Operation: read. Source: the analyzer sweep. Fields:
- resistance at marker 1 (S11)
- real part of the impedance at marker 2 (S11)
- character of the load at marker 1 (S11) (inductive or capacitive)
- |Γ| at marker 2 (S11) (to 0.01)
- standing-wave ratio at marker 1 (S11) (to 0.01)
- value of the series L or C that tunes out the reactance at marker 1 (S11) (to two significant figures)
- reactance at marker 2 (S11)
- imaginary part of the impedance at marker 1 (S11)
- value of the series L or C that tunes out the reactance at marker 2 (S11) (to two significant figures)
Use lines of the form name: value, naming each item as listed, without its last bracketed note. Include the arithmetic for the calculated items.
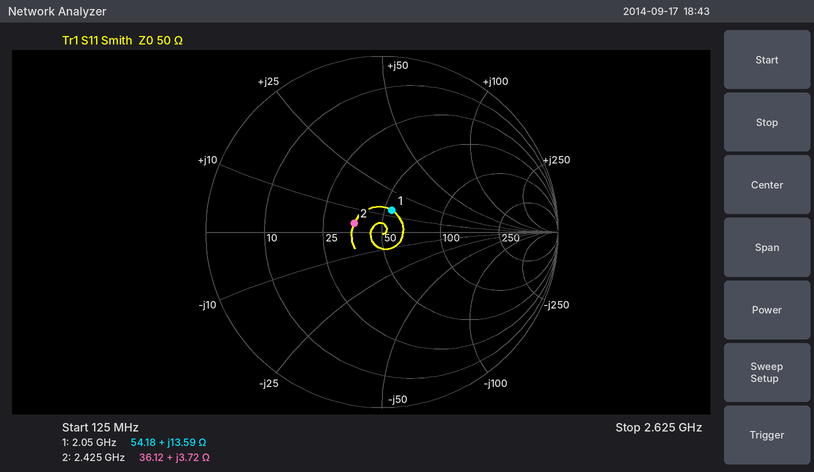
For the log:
resistance at marker 1: 54.18 Ω
real part of the impedance at marker 2: 36.12 Ω
character of the load at marker 1 (S11): inductive
|Γ| at marker 2 (S11): 0.17
standing-wave ratio at marker 1 (S11): 1.31
value of the series L or C that tunes out the reactance at marker 1 (S11): C = 1/(2π × 2.05 GHz × 13.59 Ω) ≈ 5.7 pF
reactance at marker 2: +3.72 Ω
imaginary part of the impedance at marker 1: +13.59 Ω
value of the series L or C that tunes out the reactance at marker 2 (S11): C = 1/(2π × 2.425 GHz × 3.72 Ω) ≈ 18 pF
